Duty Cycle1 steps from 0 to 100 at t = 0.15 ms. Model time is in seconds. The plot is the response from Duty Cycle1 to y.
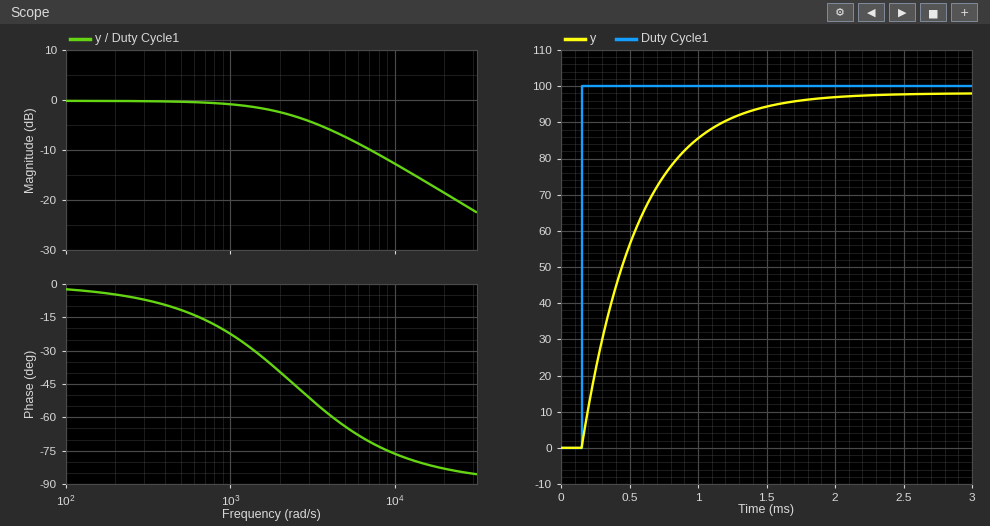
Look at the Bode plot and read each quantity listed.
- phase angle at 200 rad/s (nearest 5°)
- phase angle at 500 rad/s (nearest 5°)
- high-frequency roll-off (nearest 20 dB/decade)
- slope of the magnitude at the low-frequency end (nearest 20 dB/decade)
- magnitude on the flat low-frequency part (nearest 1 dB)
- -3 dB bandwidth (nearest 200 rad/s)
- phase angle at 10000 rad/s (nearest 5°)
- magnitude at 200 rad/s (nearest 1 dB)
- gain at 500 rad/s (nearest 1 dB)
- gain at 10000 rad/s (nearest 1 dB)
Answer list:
-5°
-10°
-20 dB/decade
0 dB/decade
0 dB
2400 rad/s
-75°
0 dB
0 dB
-13 dB
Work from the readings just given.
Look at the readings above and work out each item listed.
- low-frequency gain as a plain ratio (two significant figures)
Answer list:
1.0
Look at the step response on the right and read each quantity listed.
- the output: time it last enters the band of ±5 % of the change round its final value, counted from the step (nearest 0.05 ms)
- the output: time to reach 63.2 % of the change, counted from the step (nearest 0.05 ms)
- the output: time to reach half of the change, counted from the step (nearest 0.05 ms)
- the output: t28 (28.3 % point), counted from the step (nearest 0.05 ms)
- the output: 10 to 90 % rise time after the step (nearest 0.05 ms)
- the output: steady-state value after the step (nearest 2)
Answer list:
1.25 ms
0.40 ms
0.30 ms
0.15 ms
0.90 ms
98
